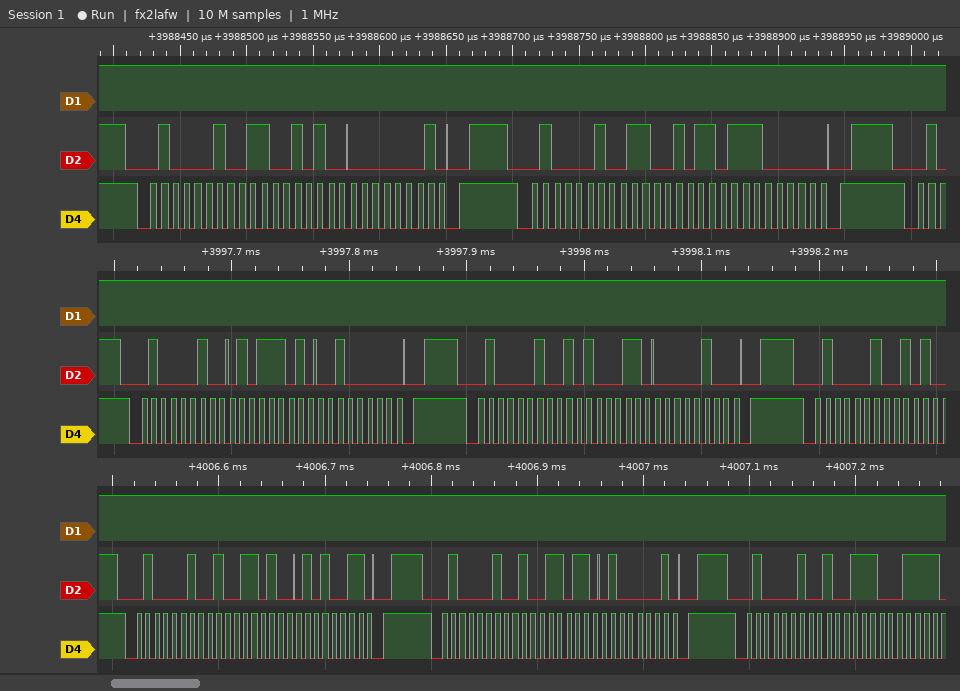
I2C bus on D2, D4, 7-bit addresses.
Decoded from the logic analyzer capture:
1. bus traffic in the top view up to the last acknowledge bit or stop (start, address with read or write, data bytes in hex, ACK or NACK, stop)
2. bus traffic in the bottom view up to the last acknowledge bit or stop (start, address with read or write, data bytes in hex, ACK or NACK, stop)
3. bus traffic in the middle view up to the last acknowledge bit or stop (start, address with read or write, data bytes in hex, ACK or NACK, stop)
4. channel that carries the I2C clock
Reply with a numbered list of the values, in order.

1. start, address 21 write ACK, CA ACK, 01 ACK, stop, start, address 21 write ACK, CB ACK, E0 ACK, stop
2. start, address 21 write ACK, 9A ACK, 53 ACK, stop, start, address 21 write ACK, 9B ACK, 41 ACK, stop, start, address 21 write ACK, 9C ACK
3. start, address 21 write ACK, 5D ACK, 20 ACK, stop, start, address 21 write ACK, A3 ACK, 04 ACK, stop, start, address 21 write ACK
4. D4
